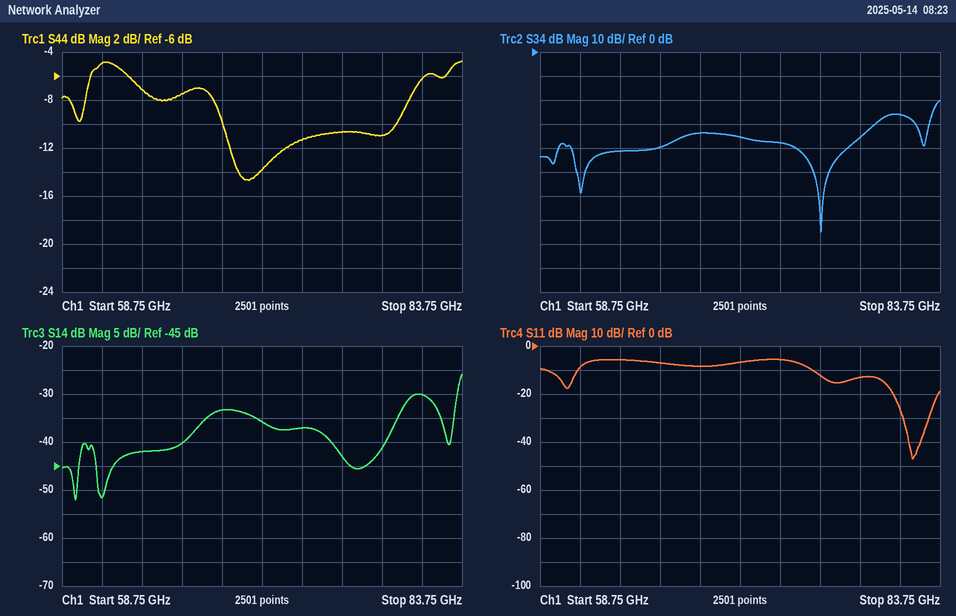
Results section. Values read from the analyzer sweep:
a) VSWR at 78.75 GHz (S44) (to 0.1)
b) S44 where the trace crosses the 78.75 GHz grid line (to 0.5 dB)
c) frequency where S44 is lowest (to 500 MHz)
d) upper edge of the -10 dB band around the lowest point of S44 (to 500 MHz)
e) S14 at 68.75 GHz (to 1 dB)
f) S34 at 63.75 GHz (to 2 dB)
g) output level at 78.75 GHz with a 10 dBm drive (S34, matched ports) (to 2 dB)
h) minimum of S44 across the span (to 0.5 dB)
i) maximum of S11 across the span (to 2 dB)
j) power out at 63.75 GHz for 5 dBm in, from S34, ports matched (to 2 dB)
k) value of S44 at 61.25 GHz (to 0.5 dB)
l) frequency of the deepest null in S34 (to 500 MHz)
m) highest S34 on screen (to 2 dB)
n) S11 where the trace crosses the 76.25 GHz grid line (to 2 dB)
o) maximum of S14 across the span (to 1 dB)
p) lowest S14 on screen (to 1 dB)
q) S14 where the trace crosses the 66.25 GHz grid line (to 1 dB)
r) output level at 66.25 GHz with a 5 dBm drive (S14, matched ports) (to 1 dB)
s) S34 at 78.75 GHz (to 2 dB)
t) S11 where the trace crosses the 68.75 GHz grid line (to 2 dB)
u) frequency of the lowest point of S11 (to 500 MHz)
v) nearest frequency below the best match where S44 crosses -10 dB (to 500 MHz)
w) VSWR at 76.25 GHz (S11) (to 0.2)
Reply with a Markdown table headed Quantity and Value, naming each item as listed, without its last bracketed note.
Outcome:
| Quantity | Value |
|---|---|
| VSWR at 78.75 GHz (S44) | 1.8 |
| S44 where the trace crosses the 78.75 GHz grid line | -11.0 dB |
| frequency where S44 is lowest | 70.5 GHz |
| upper edge of the -10 dB band around the lowest point of S44 | 79.5 GHz |
| S14 at 68.75 GHz | -33 dB |
| S34 at 63.75 GHz | -42 dB |
| output level at 78.75 GHz with a 10 dBm drive (S34, matched ports) | -26 dBm |
| minimum of S44 across the span | -14.5 dB |
| maximum of S11 across the span | -6 dB |
| power out at 63.75 GHz for 5 dBm in, from S34, ports matched | -36 dBm |
| value of S44 at 61.25 GHz | -5.0 dB |
| frequency of the deepest null in S34 | 76.5 GHz |
| highest S34 on screen | -20 dB |
| S11 where the trace crosses the 76.25 GHz grid line | -12 dB |
| maximum of S14 across the span | -26 dB |
| lowest S14 on screen | -52 dB |
| S14 where the trace crosses the 66.25 GHz grid line | -40 dB |
| output level at 66.25 GHz with a 5 dBm drive (S14, matched ports) | -35 dBm |
| S34 at 78.75 GHz | -36 dB |
| S11 where the trace crosses the 68.75 GHz grid line | -8 dB |
| frequency of the lowest point of S11 | 82.0 GHz |
| nearest frequency below the best match where S44 crosses -10 dB | 69.0 GHz |
| VSWR at 76.25 GHz (S11) | 1.6 |
